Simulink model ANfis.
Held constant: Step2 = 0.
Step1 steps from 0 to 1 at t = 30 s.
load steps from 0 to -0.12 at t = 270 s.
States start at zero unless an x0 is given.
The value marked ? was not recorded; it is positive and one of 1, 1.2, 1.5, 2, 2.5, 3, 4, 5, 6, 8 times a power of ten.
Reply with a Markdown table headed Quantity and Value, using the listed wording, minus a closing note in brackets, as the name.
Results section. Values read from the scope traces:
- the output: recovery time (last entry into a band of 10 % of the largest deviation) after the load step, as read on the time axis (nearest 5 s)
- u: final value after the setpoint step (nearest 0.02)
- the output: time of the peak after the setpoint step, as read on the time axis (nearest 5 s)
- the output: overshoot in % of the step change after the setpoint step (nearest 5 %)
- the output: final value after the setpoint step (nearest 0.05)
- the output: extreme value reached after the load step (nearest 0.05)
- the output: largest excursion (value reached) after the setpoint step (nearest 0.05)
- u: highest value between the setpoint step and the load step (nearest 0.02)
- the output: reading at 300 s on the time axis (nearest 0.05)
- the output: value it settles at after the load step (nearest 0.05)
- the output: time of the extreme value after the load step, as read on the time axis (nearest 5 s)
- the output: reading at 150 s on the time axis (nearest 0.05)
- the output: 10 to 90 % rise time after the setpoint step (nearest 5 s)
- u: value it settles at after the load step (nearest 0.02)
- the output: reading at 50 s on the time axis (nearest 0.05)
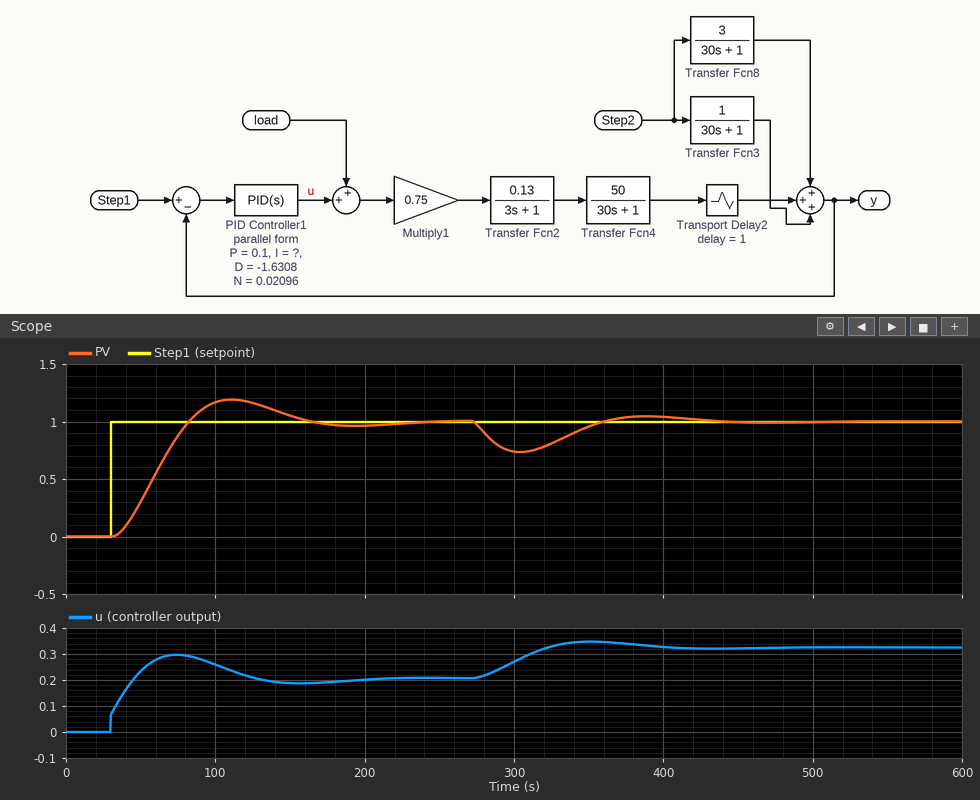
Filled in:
| Quantity | Value |
|---|---|
| the output: recovery time (last entry into a band of 10 % of the largest deviation) after the load step, as read on the time axis | 415 s |
| u: final value after the setpoint step | 0.20 |
| the output: time of the peak after the setpoint step, as read on the time axis | 110 s |
| the output: overshoot in % of the step change after the setpoint step | 20 % |
| the output: final value after the setpoint step | 1.00 |
| the output: extreme value reached after the load step | 0.75 |
| the output: largest excursion (value reached) after the setpoint step | 1.20 |
| u: highest value between the setpoint step and the load step | 0.30 |
| the output: reading at 300 s on the time axis | 0.75 |
| the output: value it settles at after the load step | 1.00 |
| the output: time of the extreme value after the load step, as read on the time axis | 305 s |
| the output: reading at 150 s on the time axis | 1.05 |
| the output: 10 to 90 % rise time after the setpoint step | 35 s |
| u: value it settles at after the load step | 0.32 |
| the output: reading at 50 s on the time axis | 0.30 |
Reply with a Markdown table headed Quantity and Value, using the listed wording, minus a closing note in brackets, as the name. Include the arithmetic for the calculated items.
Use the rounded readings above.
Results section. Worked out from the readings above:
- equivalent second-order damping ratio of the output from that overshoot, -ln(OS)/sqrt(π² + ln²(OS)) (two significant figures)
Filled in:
| Quantity | Value |
|---|---|
| equivalent second-order damping ratio of the output from that overshoot, -ln(OS)/sqrt(π² + ln²(OS)) | ln(0.2) = -1.609; 1.609 / sqrt(9.870 + 2.590) = 0.46 |
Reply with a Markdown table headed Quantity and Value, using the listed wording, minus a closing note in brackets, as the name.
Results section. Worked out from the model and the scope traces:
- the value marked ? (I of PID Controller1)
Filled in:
| Quantity | Value |
|---|---|
| the value marked ? | 0.01 |
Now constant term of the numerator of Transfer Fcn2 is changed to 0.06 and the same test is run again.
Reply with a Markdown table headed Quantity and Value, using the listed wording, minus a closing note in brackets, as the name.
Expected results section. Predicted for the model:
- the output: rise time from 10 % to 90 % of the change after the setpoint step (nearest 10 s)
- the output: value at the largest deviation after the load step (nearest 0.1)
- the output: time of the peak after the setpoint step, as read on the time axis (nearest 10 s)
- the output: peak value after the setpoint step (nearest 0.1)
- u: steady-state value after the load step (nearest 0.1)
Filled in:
| Quantity | Value |
|---|---|
| the output: rise time from 10 % to 90 % of the change after the setpoint step | 70 s |
| the output: value at the largest deviation after the load step | 0.8 |
| the output: time of the peak after the setpoint step, as read on the time axis | 170 s |
| the output: peak value after the setpoint step | 1.1 |
| u: steady-state value after the load step | 0.6 |
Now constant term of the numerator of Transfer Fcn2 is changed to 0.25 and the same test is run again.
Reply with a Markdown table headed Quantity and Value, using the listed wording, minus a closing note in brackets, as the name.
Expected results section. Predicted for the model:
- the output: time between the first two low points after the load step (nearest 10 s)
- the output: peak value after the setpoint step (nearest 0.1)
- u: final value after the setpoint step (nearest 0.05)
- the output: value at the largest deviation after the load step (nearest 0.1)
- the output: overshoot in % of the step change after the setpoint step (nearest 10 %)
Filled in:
| Quantity | Value |
|---|---|
| the output: time between the first two low points after the load step | 110 s |
| the output: peak value after the setpoint step | 1.3 |
| u: final value after the setpoint step | 0.10 |
| the output: value at the largest deviation after the load step | 0.6 |
| the output: overshoot in % of the step change after the setpoint step | 30 % |
